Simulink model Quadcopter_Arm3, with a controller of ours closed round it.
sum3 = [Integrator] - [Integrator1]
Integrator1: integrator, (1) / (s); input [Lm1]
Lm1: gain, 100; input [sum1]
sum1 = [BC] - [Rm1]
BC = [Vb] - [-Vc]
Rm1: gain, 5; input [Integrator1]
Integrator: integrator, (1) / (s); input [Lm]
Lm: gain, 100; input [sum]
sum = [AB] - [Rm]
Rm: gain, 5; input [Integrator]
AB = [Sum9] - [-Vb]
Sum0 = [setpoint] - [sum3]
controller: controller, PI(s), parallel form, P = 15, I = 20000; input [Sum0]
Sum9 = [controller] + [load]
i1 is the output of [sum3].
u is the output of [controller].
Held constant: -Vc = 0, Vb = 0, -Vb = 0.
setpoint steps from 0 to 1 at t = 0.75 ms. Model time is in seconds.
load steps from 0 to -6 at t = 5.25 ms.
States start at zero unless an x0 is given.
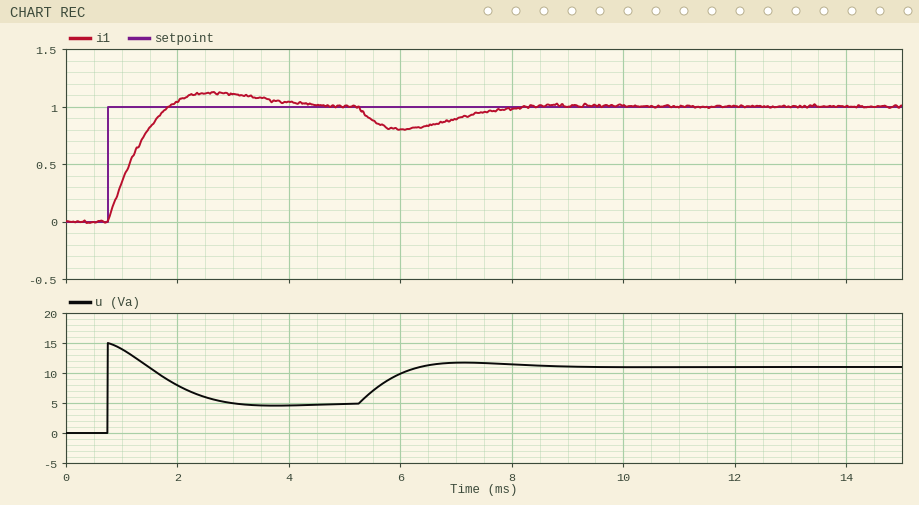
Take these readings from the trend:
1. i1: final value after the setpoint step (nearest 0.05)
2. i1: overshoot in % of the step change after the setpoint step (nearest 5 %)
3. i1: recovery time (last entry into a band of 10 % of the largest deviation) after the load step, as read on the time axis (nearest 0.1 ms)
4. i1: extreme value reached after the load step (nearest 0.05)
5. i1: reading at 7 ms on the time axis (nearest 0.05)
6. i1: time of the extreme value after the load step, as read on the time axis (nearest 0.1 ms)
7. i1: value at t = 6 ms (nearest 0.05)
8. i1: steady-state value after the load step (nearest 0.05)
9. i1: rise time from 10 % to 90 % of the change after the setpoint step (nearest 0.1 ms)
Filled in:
1.00
10 %
7.9 ms
0.80
0.90
6.0 ms
0.80
1.00
0.8 ms
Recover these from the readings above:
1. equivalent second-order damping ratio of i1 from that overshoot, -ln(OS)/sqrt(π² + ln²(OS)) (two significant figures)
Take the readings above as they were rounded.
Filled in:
0.59
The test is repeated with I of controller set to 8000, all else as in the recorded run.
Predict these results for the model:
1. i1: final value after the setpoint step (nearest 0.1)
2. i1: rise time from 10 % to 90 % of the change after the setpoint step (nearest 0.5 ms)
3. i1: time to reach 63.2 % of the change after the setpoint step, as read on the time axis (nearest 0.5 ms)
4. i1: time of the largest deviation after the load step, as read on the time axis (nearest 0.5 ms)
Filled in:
1.0
1.5 ms
1.5 ms
6.5 ms
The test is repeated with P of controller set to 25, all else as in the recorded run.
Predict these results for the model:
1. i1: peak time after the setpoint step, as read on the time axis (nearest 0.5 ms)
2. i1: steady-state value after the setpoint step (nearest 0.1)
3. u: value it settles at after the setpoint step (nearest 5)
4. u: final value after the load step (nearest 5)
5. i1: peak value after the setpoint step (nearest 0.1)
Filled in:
2.5 ms
1.0
5
10
1.0
